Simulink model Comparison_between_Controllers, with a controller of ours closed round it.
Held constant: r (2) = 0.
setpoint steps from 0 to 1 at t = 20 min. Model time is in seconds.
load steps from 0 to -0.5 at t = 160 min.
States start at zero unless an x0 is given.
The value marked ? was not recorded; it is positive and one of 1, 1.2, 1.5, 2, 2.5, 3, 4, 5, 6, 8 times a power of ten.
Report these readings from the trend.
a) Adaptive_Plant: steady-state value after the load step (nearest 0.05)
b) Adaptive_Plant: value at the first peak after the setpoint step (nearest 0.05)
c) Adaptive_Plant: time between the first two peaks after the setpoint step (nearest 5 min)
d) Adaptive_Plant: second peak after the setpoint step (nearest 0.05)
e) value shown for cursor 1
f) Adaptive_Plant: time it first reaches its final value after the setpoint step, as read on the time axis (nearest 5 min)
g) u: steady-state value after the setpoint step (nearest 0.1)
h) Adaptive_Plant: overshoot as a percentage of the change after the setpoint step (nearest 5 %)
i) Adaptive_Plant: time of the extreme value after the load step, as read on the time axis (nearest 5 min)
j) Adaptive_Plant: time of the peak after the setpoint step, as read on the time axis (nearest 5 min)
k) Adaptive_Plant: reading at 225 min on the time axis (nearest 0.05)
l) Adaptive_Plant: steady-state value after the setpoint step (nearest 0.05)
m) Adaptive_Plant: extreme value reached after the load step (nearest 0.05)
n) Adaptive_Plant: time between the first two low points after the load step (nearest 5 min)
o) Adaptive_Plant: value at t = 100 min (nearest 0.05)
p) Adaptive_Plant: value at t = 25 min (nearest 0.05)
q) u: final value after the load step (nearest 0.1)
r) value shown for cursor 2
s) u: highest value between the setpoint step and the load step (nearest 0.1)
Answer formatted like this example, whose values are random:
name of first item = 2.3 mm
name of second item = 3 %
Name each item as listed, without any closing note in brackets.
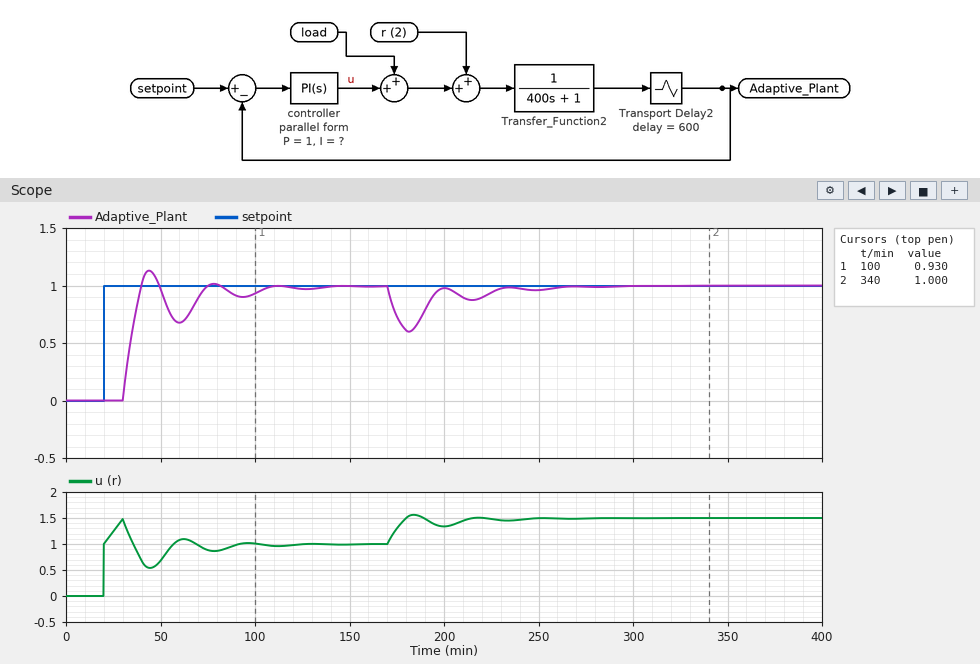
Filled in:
Adaptive_Plant: steady-state value after the load step = 1.00
Adaptive_Plant: value at the first peak after the setpoint step = 1.15
Adaptive_Plant: time between the first two peaks after the setpoint step = 35 min
Adaptive_Plant: second peak after the setpoint step = 1.00
value shown for cursor 1 = 0.930
Adaptive_Plant: time it first reaches its final value after the setpoint step, as read on the time axis = 40 min
u: steady-state value after the setpoint step = 1.0
Adaptive_Plant: overshoot as a percentage of the change after the setpoint step = 15 %
Adaptive_Plant: time of the extreme value after the load step, as read on the time axis = 180 min
Adaptive_Plant: time of the peak after the setpoint step, as read on the time axis = 45 min
Adaptive_Plant: reading at 225 min on the time axis = 0.95
Adaptive_Plant: steady-state value after the setpoint step = 1.00
Adaptive_Plant: extreme value reached after the load step = 0.60
Adaptive_Plant: time between the first two low points after the load step = 35 min
Adaptive_Plant: value at t = 100 min = 0.95
Adaptive_Plant: value at t = 25 min = 0.00
u: final value after the load step = 1.5
value shown for cursor 2 = 1.000
u: highest value between the setpoint step and the load step = 1.5
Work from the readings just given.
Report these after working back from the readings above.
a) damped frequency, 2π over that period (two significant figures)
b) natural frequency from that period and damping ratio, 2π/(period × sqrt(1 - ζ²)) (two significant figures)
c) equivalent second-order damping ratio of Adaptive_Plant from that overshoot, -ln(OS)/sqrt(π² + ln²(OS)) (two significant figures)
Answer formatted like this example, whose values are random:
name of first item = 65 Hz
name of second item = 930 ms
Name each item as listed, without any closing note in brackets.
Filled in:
damped frequency, 2π over that period = 0.18 rad/min
natural frequency from that period and damping ratio, 2π/(period × sqrt(1 - ζ²)) = 0.21 rad/min
equivalent second-order damping ratio of Adaptive_Plant from that overshoot, -ln(OS)/sqrt(π² + ln²(OS)) = 0.52
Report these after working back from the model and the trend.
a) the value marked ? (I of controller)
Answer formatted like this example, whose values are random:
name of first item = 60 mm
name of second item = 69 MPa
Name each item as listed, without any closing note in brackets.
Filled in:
the value marked ? = 0.0008
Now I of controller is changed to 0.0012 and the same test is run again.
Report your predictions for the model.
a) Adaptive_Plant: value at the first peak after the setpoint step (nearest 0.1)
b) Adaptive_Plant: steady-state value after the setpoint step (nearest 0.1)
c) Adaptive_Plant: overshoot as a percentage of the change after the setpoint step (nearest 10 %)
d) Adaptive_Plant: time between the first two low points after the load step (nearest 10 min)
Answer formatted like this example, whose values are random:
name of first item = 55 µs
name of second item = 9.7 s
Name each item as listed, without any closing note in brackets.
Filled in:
Adaptive_Plant: value at the first peak after the setpoint step = 1.3
Adaptive_Plant: steady-state value after the setpoint step = 1.0
Adaptive_Plant: overshoot as a percentage of the change after the setpoint step = 30 %
Adaptive_Plant: time between the first two low points after the load step = 40 min
